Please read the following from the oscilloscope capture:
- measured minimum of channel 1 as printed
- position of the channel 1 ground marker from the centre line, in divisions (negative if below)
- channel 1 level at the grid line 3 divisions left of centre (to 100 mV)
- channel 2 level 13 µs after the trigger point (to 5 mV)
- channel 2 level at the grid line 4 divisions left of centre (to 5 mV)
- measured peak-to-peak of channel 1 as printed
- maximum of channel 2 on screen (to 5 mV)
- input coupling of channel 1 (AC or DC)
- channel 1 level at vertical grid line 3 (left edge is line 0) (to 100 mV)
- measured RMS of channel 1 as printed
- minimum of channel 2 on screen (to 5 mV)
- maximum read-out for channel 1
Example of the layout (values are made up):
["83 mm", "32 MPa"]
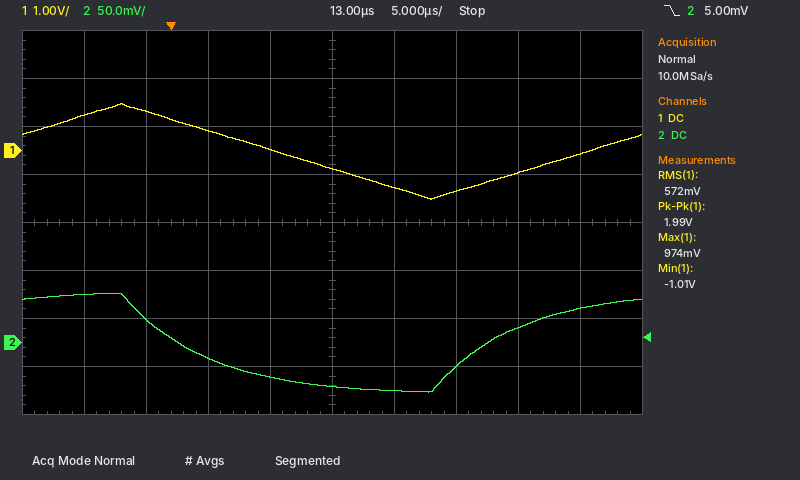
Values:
["-1.01 V", "+1.5 div", "800 mV", "-45 mV", "50 mV", "1.99 V", "50 mV", "DC", "400 mV", "572 mV", "-50 mV", "974 mV"]
